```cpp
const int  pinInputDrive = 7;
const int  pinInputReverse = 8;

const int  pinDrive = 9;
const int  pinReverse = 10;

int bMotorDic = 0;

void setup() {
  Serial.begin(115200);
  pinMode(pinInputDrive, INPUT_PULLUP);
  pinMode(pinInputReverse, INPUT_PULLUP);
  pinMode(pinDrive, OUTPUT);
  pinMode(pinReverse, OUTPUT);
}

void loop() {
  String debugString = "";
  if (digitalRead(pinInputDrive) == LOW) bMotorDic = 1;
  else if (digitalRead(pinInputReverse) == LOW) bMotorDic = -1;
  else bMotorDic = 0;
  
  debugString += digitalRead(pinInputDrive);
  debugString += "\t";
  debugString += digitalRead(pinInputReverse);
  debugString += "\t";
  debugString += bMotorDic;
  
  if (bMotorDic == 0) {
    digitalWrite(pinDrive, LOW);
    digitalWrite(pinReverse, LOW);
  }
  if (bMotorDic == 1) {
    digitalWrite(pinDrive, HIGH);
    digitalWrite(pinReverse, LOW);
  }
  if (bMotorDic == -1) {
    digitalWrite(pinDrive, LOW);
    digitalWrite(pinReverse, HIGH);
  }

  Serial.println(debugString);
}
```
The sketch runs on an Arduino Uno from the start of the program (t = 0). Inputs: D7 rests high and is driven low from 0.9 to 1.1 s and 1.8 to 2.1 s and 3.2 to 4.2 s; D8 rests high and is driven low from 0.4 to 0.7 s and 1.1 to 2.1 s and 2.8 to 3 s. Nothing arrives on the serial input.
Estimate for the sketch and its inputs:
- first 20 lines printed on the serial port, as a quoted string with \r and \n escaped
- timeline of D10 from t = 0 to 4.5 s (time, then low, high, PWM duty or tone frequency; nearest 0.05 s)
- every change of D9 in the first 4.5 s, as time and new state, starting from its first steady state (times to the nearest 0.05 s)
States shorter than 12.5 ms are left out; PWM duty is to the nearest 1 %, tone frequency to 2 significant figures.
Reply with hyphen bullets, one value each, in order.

- "1\t1\t0\r\n1\t1\t0\r\n1\t1\t0\r\n1\t1\t0\r\n1\t1\t0\r\n1\t1\t0\r\n1\t1\t0\r\n1\t1\t0\r\n1\t1\t0\r\n1\t1\t0\r\n1\t1\t0\r\n1\t1\t0\r\n1\t1\t0\r\n1\t1\t0\r\n1\t1\t0\r\n1\t1\t0\r\n1\t1\t0\r\n1\t1\t0\r\n1\t1\t0\r\n1\t1\t0\r\n"
- 0 s low; 0.4 s high; 0.7 s low; 1.1 s high; 1.8 s low; 2.8 s high; 3 s low
- 0 s low; 0.9 s high; 1.1 s low; 1.8 s high; 2.1 s low; 3.2 s high; 4.2 s low
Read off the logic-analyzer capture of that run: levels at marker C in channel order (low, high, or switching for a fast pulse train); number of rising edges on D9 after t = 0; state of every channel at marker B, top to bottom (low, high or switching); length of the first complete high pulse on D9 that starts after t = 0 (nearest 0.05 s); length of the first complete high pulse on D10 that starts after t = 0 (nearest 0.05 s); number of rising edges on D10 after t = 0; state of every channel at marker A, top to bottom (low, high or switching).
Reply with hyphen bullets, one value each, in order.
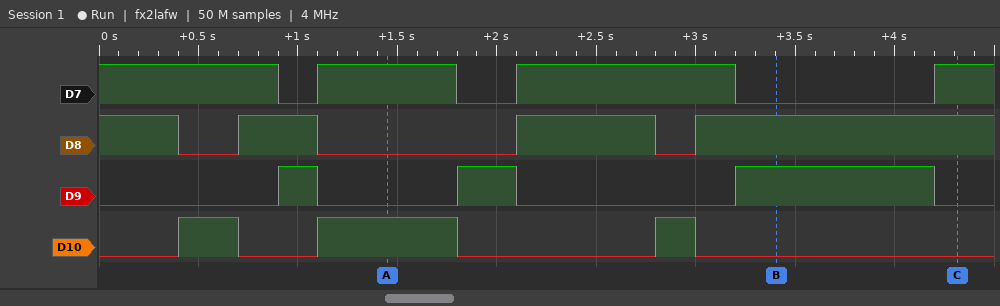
- D7 high, D8 high, D9 low, D10 low
- 3
- D7 low, D8 high, D9 high, D10 low
- 0.20 s
- 0.30 s
- 3
- D7 high, D8 low, D9 low, D10 high
